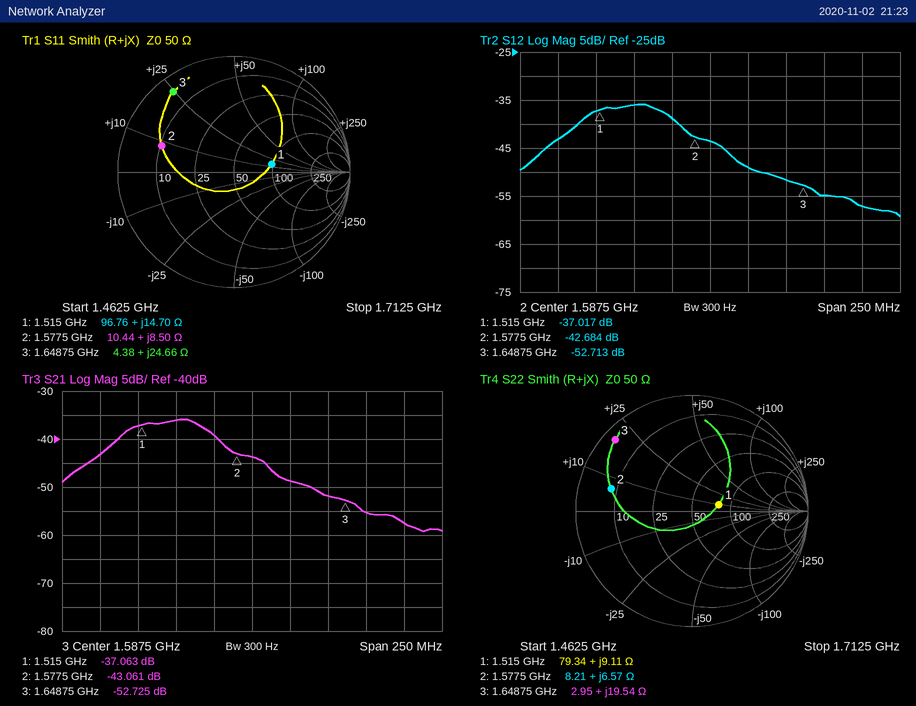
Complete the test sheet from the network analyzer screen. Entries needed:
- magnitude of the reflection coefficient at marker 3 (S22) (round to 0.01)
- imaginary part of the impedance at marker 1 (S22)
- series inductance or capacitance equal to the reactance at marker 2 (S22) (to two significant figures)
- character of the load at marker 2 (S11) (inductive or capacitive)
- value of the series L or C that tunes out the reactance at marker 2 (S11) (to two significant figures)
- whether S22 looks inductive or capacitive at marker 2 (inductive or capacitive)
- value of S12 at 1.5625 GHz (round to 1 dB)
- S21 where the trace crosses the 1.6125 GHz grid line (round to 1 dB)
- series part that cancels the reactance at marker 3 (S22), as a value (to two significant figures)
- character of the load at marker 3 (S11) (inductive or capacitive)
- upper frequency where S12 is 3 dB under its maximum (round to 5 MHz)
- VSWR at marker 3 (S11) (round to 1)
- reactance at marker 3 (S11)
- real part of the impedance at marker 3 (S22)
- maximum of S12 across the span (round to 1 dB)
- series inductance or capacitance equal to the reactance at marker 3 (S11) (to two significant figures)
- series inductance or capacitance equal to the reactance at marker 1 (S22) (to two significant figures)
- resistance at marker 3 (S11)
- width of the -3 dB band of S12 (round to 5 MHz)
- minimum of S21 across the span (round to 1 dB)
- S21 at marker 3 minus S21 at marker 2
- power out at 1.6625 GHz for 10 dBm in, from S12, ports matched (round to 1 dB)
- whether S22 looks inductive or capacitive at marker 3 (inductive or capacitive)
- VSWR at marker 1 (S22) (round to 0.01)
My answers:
0.90
+9.11 Ω
660 pH
inductive
12 pF
inductive
-39 dB
-49 dB
4.9 pF
inductive
1.565 GHz
14
+24.66 Ω
2.95 Ω
-36 dB
2.4 nH
960 pH
4.38 Ω
60 MHz
-59 dB
-9.664 dB
-45 dBm
inductive
1.62
